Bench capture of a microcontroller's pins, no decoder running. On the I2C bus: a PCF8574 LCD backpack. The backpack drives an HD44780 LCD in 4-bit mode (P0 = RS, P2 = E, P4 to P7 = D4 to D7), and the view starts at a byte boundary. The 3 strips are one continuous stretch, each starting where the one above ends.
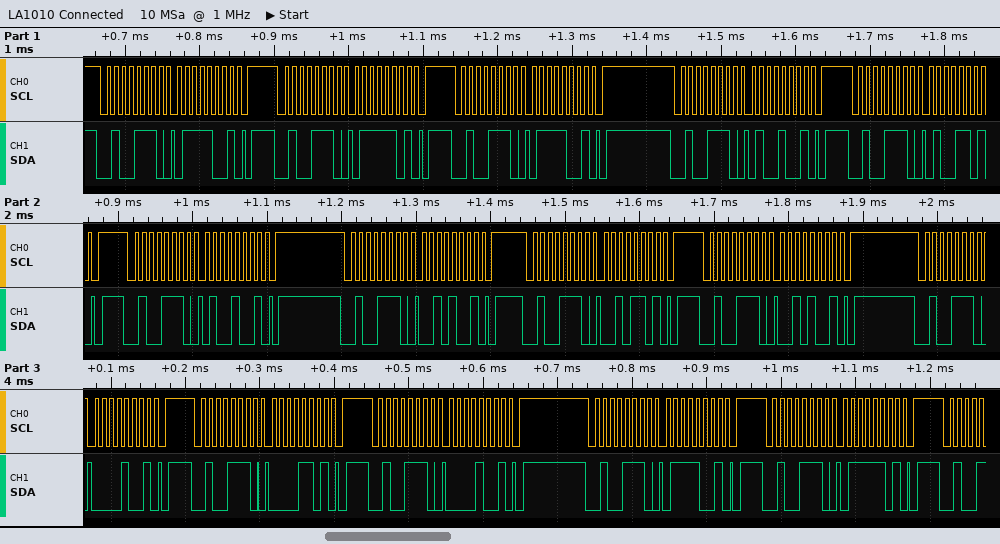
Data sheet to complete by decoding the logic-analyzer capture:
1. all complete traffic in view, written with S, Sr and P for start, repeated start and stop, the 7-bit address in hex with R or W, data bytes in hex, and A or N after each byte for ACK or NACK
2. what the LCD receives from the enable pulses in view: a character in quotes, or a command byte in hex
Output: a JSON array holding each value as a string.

["S 27W A 79 A P S 27W A 7D A P S 27W A 79 A P S 27W A 49 A P S 27W A 4D A P S 27W A 49 A P S 27W A 29 A P S 27W A 2D A P S 27W A 29 A P S 27W A 09 A P S 27W A 0D A P S 27W A 09 A P S 27W A 79 A P S 27W A 7D A P", "'t' ' '"]
